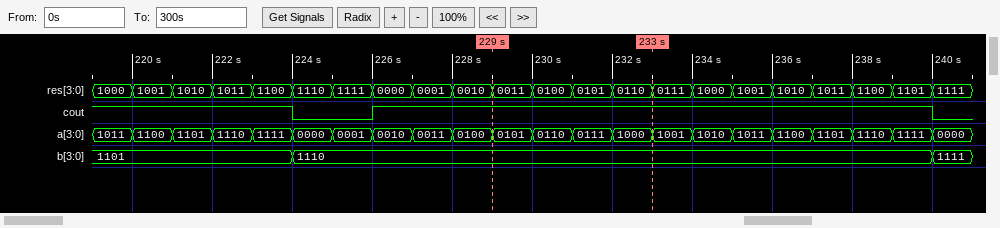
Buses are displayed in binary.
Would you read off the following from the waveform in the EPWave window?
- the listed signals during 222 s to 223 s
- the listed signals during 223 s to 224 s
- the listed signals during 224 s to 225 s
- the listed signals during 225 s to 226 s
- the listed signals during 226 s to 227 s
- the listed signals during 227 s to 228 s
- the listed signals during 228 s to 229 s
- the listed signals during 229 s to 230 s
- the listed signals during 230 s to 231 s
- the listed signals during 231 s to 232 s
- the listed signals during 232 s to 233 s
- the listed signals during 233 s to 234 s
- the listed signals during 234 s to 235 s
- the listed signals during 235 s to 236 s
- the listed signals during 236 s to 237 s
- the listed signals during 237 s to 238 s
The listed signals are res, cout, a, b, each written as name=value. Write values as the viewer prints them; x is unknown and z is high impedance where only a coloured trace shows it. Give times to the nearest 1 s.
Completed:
res=1011, cout=1, a=1110, b=1101
res=1100, cout=1, a=1111, b=1101
res=1110, cout=0, a=0000, b=1110
res=1111, cout=0, a=0001, b=1110
res=0000, cout=1, a=0010, b=1110
res=0001, cout=1, a=0011, b=1110
res=0010, cout=1, a=0100, b=1110
res=0011, cout=1, a=0101, b=1110
res=0100, cout=1, a=0110, b=1110
res=0101, cout=1, a=0111, b=1110
res=0110, cout=1, a=1000, b=1110
res=0111, cout=1, a=1001, b=1110
res=1000, cout=1, a=1010, b=1110
res=1001, cout=1, a=1011, b=1110
res=1010, cout=1, a=1100, b=1110
res=1011, cout=1, a=1101, b=1110
